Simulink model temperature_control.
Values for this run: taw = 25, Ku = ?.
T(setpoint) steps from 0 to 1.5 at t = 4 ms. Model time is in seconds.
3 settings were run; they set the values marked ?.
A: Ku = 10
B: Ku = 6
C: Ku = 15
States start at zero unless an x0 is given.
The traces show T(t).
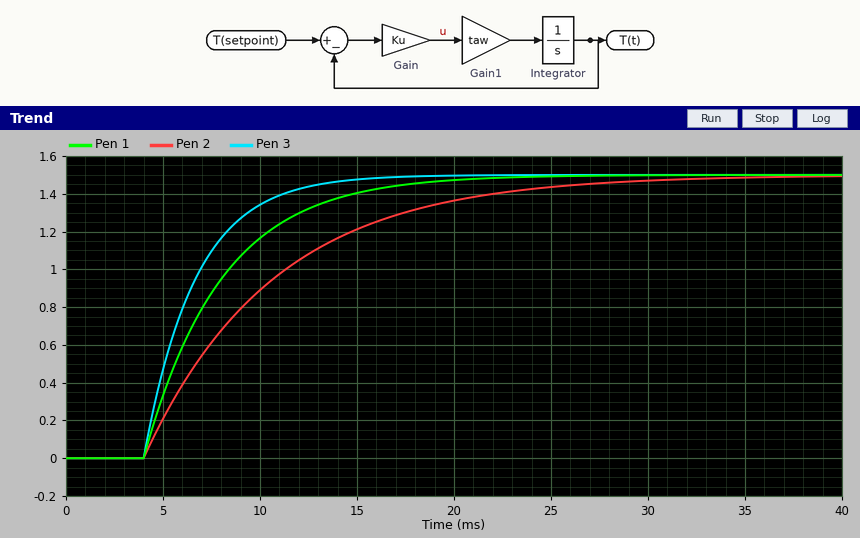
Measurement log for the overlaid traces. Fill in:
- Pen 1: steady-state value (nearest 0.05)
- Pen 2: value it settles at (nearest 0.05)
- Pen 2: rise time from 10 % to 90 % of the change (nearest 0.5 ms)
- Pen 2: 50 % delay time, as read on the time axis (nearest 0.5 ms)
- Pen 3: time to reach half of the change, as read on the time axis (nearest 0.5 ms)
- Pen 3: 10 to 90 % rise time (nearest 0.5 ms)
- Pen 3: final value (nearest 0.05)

1.50
1.50
14.5 ms
8.5 ms
6.0 ms
6.0 ms
1.50
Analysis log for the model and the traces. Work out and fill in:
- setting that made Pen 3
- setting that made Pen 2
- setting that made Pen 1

C
B
A
